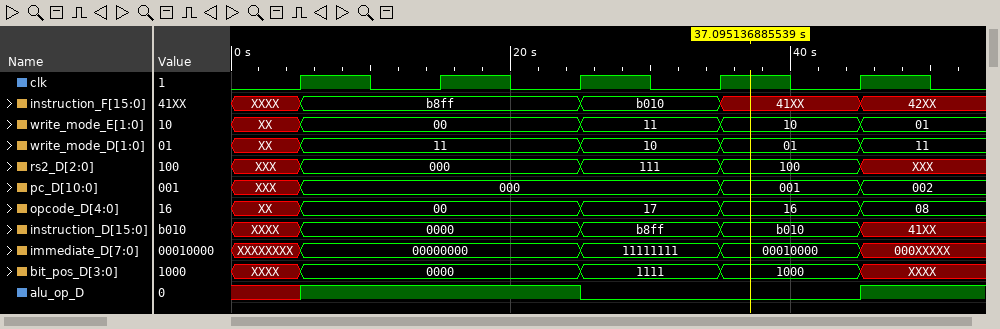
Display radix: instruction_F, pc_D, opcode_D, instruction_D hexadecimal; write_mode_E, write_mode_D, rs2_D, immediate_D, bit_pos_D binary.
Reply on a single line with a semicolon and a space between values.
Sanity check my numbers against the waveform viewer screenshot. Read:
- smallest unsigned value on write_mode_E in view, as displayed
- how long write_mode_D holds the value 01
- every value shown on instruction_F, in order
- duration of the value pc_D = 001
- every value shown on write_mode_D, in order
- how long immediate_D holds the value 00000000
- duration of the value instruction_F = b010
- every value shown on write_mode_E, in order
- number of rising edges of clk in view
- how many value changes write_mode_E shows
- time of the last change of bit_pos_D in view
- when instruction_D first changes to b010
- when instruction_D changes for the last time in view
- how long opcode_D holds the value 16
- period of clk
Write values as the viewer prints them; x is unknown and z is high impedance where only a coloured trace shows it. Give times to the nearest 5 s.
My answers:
00; 10 s; XXXX, b8ff, b010, 41XX, 42XX; 10 s; XX, 11, 10, 01, 11; 20 s; 10 s; XX, 00, 11, 10, 01; 5; 4; 45 s; 35 s; 45 s; 10 s; 10 s
